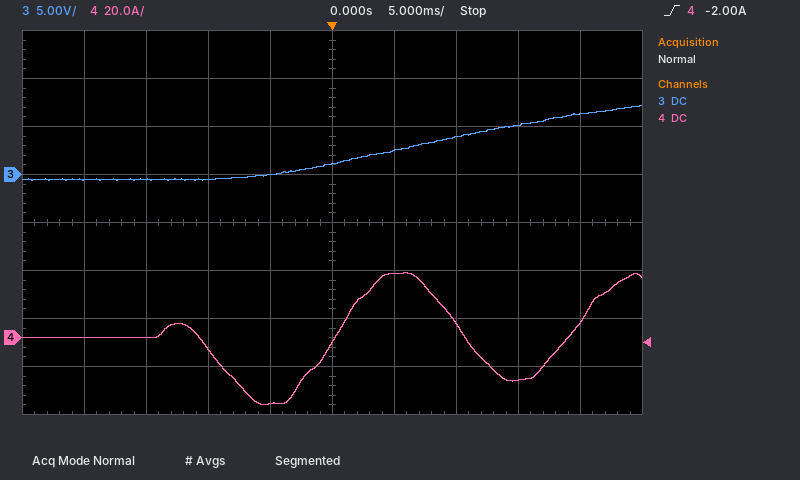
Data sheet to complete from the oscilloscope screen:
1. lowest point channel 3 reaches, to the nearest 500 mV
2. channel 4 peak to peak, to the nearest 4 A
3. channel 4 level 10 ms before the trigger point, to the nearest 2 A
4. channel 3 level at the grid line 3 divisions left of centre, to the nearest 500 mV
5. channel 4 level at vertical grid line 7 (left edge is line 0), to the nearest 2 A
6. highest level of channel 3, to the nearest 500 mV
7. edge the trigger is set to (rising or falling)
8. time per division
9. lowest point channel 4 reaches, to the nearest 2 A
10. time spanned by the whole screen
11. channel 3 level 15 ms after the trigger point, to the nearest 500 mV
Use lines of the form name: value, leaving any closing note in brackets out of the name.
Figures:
lowest point channel 3 reaches, to the nearest 500 mV: -500 mV
channel 4 peak to peak, to the nearest 4 A: 56 A
channel 4 level 10 ms before the trigger point, to the nearest 2 A: -4 A
channel 3 level at the grid line 3 divisions left of centre, to the nearest 500 mV: -500 mV
channel 4 level at vertical grid line 7 (left edge is line 0), to the nearest 2 A: 6 A
highest level of channel 3, to the nearest 500 mV: 7.0 V
edge the trigger is set to: rising
time per division: 5 ms
lowest point channel 4 reaches, to the nearest 2 A: -28 A
time spanned by the whole screen: 50 ms
channel 3 level 15 ms after the trigger point, to the nearest 500 mV: 5.0 V
